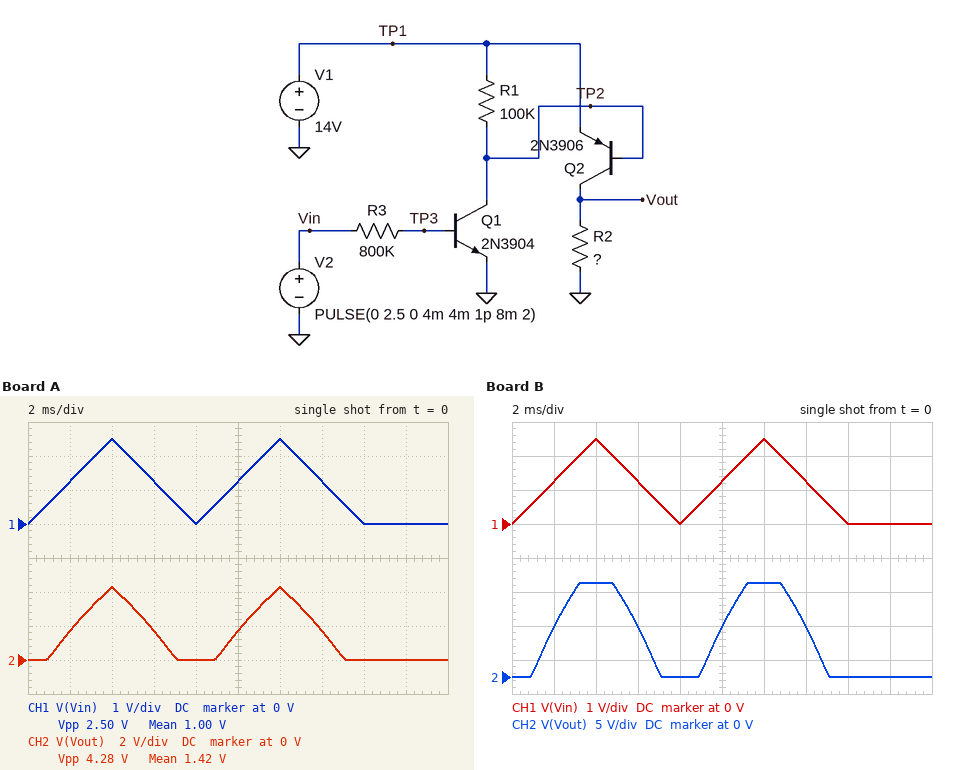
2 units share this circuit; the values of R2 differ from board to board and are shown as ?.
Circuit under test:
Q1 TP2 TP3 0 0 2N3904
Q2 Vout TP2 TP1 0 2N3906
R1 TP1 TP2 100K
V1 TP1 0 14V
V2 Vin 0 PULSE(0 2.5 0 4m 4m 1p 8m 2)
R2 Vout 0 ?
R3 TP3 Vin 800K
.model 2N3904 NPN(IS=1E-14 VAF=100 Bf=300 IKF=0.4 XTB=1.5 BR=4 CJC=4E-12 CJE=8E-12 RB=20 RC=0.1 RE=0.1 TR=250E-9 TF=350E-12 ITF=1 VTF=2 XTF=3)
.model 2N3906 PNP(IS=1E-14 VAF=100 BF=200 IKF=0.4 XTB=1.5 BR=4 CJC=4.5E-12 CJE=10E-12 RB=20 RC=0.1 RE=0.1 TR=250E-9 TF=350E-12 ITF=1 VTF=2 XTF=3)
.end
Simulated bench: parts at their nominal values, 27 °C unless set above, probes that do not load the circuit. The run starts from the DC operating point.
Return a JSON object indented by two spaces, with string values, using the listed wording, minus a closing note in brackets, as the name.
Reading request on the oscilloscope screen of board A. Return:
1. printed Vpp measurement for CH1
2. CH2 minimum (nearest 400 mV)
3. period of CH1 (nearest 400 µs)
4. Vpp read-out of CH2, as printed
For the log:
{
  "printed Vpp measurement for CH1": "2.50 V",
  "CH2 minimum": "0 V",
  "period of CH1": "8.0 ms",
  "Vpp read-out of CH2, as printed": "4.28 V"
}
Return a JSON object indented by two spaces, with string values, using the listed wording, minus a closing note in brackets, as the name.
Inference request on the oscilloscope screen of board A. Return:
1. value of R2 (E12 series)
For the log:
{
  "value of R2": "33 Ω"
}
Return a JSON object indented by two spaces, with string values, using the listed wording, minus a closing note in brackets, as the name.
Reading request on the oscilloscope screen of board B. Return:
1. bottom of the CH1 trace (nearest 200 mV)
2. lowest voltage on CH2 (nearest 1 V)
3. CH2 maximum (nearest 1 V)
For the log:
{
  "bottom of the CH1 trace": "0 V",
  "lowest voltage on CH2": "0 V",
  "CH2 maximum": "14 V"
}
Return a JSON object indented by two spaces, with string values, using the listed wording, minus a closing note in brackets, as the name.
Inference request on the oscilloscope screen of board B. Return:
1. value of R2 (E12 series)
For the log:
{
  "value of R2": "150 Ω"
}
